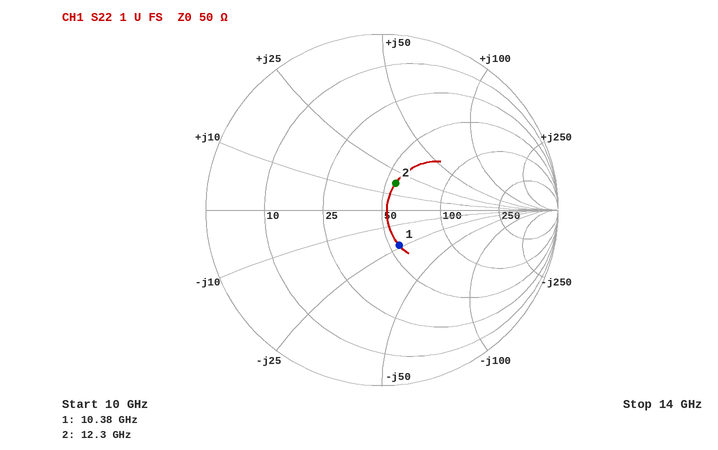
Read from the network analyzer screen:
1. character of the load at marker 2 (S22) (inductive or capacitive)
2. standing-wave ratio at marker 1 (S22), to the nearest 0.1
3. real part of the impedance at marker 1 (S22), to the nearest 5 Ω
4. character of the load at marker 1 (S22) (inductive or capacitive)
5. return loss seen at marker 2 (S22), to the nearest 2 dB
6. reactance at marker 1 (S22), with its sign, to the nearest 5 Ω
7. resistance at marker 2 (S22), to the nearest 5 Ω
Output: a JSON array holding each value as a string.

["inductive", "1.6", "55 Ω", "capacitive", "16 dB", "-25 Ω", "55 Ω"]
